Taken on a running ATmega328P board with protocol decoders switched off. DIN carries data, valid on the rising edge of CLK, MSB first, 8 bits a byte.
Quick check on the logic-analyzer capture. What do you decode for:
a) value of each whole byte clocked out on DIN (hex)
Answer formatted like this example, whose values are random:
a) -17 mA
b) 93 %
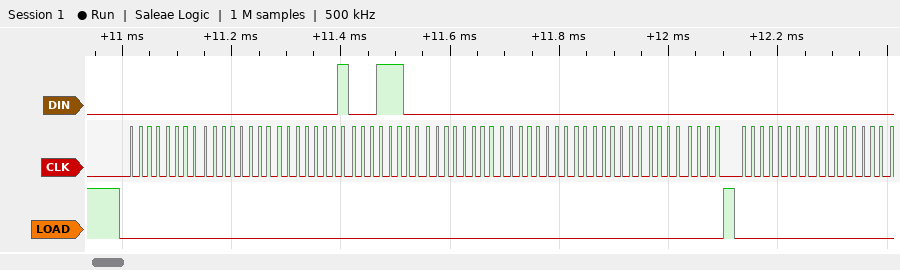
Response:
a) 00 00 01 1C 00 00 00 00 00 00
